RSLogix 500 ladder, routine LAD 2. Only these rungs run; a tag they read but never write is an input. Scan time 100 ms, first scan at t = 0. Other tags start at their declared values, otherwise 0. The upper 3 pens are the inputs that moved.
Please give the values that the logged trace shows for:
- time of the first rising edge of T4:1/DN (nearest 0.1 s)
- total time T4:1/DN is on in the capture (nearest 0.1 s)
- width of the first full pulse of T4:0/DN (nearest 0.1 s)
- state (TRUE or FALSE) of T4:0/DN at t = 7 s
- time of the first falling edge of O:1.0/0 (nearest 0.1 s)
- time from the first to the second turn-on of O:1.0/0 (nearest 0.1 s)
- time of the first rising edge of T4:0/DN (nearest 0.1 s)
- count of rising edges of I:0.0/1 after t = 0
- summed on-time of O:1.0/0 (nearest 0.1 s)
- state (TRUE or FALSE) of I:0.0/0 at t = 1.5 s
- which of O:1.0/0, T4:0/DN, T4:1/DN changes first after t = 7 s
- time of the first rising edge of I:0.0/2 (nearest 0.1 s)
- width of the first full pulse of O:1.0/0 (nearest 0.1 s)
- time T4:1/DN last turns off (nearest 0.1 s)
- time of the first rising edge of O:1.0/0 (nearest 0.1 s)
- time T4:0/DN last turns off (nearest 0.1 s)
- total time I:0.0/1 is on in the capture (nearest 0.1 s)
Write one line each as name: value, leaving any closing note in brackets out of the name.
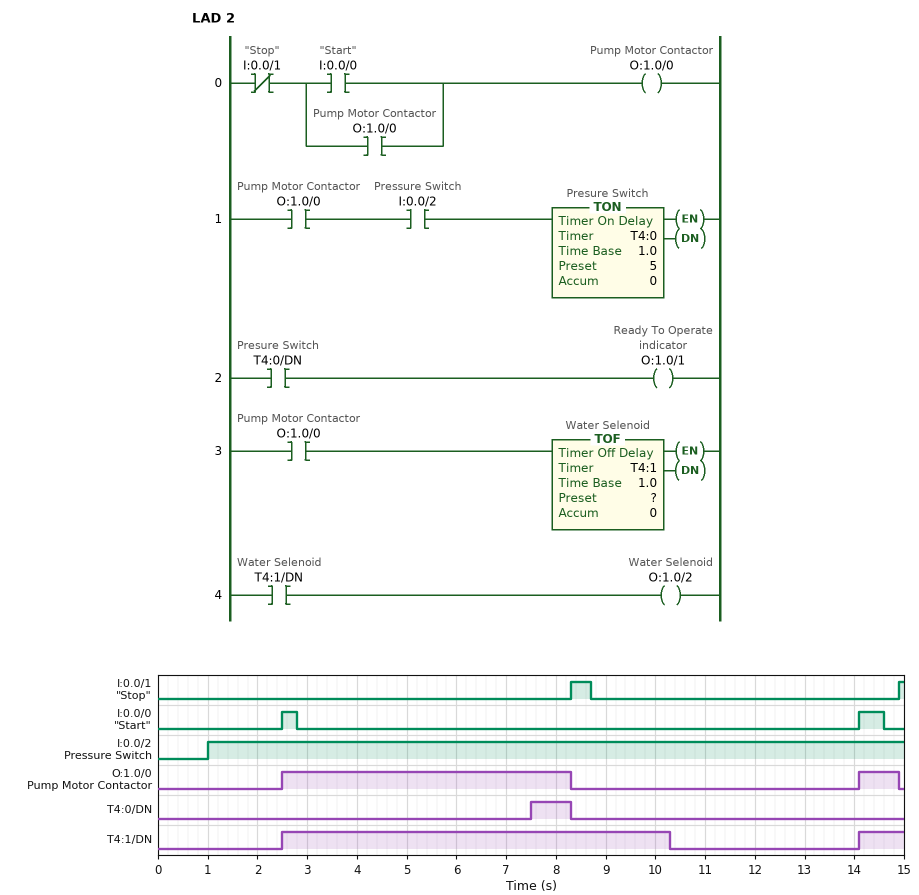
time of the first rising edge of T4:1/DN: 2.5 s
total time T4:1/DN is on in the capture: 8.7 s
width of the first full pulse of T4:0/DN: 0.8 s
state (TRUE or FALSE) of T4:0/DN at t = 7 s: FALSE
time of the first falling edge of O:1.0/0: 8.3 s
time from the first to the second turn-on of O:1.0/0: 11.6 s
time of the first rising edge of T4:0/DN: 7.5 s
count of rising edges of I:0.0/1 after t = 0: 2
summed on-time of O:1.0/0: 6.6 s
state (TRUE or FALSE) of I:0.0/0 at t = 1.5 s: FALSE
which of O:1.0/0, T4:0/DN, T4:1/DN changes first after t = 7 s: T4:0/DN
time of the first rising edge of I:0.0/2: 1.0 s
width of the first full pulse of O:1.0/0: 5.8 s
time T4:1/DN last turns off: 10.3 s
time of the first rising edge of O:1.0/0: 2.5 s
time T4:0/DN last turns off: 8.3 s
total time I:0.0/1 is on in the capture: 0.5 s
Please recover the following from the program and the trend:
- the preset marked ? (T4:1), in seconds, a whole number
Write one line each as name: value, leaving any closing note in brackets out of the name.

the preset marked ? (T4:1), in seconds, a whole number: 2 s
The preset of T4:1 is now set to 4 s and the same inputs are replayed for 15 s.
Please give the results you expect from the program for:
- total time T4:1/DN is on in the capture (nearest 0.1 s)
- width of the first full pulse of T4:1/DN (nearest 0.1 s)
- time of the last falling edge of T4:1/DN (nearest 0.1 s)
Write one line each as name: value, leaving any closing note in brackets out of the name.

total time T4:1/DN is on in the capture: 10.7 s
width of the first full pulse of T4:1/DN: 9.8 s
time of the last falling edge of T4:1/DN: 12.3 s
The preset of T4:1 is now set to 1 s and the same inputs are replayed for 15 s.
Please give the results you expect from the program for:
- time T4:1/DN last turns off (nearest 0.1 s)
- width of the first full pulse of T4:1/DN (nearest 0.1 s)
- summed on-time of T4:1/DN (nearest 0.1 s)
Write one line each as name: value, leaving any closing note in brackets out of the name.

time T4:1/DN last turns off: 9.3 s
width of the first full pulse of T4:1/DN: 6.8 s
summed on-time of T4:1/DN: 7.7 s
